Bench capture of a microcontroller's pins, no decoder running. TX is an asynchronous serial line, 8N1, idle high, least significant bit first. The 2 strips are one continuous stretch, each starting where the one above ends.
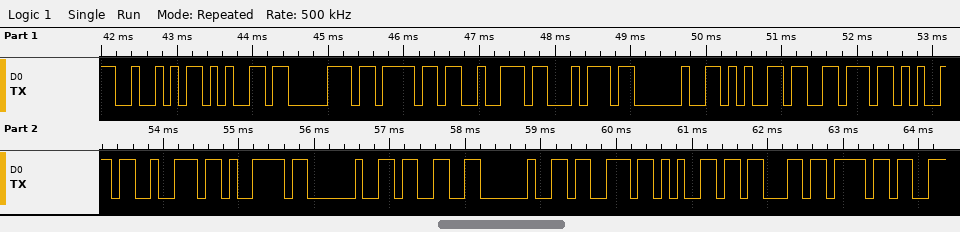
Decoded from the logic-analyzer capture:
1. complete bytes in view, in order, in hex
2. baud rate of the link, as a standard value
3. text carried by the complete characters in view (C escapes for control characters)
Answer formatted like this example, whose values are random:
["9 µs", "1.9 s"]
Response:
["52 65 70 6F 72 74 20 65 76 65 72 79 20 33 20 73 65 63 6F", "9600 baud", "\"Report every 3 seco\""]
